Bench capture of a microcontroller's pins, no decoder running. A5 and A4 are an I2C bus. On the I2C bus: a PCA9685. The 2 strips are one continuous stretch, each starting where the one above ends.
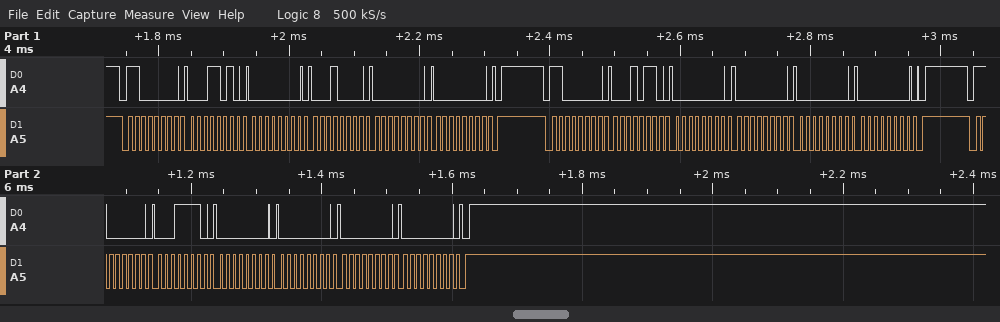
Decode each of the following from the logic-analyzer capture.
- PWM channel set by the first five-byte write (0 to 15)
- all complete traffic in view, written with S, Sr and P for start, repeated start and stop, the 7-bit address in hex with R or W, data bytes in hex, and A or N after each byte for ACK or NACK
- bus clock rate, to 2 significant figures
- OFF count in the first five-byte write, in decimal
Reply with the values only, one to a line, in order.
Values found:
5
S 60W A 1A A 00 A 10 A 00 A 00 A P S 60W A 16 A 00 A 00 A 00 A 00 A P S 60W A 1E A 00 A 00 A 00 A 00 A P
100 kHz
0
